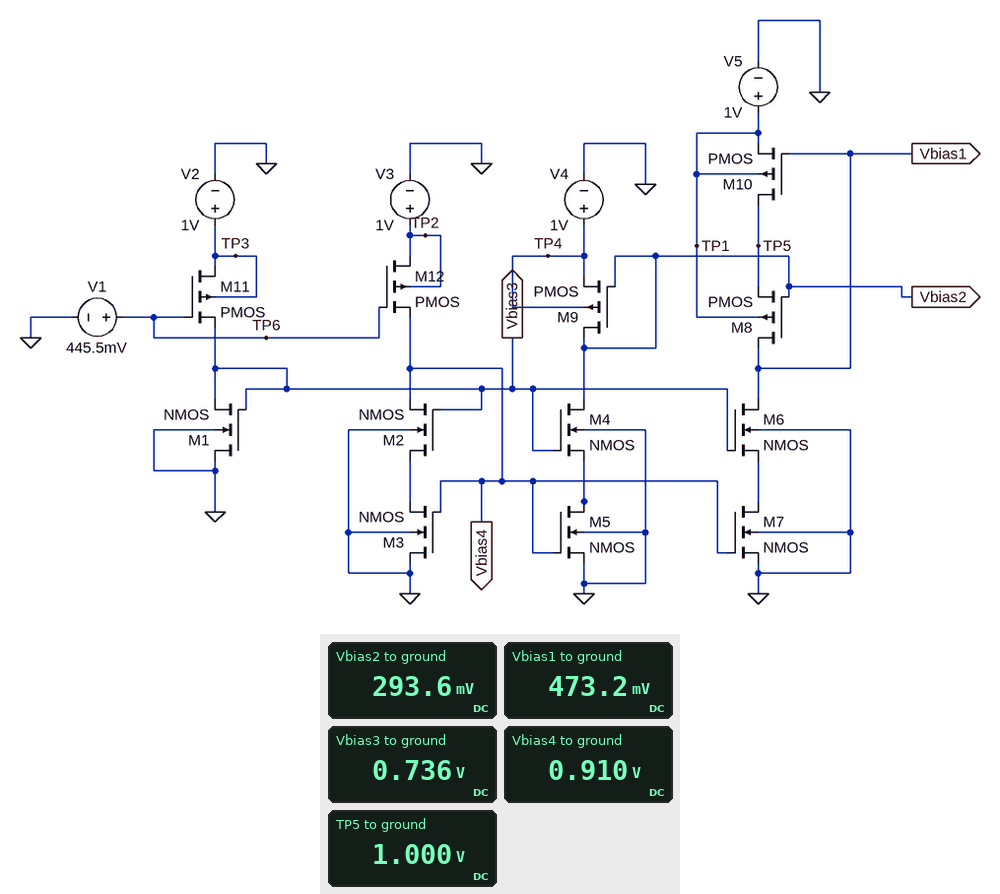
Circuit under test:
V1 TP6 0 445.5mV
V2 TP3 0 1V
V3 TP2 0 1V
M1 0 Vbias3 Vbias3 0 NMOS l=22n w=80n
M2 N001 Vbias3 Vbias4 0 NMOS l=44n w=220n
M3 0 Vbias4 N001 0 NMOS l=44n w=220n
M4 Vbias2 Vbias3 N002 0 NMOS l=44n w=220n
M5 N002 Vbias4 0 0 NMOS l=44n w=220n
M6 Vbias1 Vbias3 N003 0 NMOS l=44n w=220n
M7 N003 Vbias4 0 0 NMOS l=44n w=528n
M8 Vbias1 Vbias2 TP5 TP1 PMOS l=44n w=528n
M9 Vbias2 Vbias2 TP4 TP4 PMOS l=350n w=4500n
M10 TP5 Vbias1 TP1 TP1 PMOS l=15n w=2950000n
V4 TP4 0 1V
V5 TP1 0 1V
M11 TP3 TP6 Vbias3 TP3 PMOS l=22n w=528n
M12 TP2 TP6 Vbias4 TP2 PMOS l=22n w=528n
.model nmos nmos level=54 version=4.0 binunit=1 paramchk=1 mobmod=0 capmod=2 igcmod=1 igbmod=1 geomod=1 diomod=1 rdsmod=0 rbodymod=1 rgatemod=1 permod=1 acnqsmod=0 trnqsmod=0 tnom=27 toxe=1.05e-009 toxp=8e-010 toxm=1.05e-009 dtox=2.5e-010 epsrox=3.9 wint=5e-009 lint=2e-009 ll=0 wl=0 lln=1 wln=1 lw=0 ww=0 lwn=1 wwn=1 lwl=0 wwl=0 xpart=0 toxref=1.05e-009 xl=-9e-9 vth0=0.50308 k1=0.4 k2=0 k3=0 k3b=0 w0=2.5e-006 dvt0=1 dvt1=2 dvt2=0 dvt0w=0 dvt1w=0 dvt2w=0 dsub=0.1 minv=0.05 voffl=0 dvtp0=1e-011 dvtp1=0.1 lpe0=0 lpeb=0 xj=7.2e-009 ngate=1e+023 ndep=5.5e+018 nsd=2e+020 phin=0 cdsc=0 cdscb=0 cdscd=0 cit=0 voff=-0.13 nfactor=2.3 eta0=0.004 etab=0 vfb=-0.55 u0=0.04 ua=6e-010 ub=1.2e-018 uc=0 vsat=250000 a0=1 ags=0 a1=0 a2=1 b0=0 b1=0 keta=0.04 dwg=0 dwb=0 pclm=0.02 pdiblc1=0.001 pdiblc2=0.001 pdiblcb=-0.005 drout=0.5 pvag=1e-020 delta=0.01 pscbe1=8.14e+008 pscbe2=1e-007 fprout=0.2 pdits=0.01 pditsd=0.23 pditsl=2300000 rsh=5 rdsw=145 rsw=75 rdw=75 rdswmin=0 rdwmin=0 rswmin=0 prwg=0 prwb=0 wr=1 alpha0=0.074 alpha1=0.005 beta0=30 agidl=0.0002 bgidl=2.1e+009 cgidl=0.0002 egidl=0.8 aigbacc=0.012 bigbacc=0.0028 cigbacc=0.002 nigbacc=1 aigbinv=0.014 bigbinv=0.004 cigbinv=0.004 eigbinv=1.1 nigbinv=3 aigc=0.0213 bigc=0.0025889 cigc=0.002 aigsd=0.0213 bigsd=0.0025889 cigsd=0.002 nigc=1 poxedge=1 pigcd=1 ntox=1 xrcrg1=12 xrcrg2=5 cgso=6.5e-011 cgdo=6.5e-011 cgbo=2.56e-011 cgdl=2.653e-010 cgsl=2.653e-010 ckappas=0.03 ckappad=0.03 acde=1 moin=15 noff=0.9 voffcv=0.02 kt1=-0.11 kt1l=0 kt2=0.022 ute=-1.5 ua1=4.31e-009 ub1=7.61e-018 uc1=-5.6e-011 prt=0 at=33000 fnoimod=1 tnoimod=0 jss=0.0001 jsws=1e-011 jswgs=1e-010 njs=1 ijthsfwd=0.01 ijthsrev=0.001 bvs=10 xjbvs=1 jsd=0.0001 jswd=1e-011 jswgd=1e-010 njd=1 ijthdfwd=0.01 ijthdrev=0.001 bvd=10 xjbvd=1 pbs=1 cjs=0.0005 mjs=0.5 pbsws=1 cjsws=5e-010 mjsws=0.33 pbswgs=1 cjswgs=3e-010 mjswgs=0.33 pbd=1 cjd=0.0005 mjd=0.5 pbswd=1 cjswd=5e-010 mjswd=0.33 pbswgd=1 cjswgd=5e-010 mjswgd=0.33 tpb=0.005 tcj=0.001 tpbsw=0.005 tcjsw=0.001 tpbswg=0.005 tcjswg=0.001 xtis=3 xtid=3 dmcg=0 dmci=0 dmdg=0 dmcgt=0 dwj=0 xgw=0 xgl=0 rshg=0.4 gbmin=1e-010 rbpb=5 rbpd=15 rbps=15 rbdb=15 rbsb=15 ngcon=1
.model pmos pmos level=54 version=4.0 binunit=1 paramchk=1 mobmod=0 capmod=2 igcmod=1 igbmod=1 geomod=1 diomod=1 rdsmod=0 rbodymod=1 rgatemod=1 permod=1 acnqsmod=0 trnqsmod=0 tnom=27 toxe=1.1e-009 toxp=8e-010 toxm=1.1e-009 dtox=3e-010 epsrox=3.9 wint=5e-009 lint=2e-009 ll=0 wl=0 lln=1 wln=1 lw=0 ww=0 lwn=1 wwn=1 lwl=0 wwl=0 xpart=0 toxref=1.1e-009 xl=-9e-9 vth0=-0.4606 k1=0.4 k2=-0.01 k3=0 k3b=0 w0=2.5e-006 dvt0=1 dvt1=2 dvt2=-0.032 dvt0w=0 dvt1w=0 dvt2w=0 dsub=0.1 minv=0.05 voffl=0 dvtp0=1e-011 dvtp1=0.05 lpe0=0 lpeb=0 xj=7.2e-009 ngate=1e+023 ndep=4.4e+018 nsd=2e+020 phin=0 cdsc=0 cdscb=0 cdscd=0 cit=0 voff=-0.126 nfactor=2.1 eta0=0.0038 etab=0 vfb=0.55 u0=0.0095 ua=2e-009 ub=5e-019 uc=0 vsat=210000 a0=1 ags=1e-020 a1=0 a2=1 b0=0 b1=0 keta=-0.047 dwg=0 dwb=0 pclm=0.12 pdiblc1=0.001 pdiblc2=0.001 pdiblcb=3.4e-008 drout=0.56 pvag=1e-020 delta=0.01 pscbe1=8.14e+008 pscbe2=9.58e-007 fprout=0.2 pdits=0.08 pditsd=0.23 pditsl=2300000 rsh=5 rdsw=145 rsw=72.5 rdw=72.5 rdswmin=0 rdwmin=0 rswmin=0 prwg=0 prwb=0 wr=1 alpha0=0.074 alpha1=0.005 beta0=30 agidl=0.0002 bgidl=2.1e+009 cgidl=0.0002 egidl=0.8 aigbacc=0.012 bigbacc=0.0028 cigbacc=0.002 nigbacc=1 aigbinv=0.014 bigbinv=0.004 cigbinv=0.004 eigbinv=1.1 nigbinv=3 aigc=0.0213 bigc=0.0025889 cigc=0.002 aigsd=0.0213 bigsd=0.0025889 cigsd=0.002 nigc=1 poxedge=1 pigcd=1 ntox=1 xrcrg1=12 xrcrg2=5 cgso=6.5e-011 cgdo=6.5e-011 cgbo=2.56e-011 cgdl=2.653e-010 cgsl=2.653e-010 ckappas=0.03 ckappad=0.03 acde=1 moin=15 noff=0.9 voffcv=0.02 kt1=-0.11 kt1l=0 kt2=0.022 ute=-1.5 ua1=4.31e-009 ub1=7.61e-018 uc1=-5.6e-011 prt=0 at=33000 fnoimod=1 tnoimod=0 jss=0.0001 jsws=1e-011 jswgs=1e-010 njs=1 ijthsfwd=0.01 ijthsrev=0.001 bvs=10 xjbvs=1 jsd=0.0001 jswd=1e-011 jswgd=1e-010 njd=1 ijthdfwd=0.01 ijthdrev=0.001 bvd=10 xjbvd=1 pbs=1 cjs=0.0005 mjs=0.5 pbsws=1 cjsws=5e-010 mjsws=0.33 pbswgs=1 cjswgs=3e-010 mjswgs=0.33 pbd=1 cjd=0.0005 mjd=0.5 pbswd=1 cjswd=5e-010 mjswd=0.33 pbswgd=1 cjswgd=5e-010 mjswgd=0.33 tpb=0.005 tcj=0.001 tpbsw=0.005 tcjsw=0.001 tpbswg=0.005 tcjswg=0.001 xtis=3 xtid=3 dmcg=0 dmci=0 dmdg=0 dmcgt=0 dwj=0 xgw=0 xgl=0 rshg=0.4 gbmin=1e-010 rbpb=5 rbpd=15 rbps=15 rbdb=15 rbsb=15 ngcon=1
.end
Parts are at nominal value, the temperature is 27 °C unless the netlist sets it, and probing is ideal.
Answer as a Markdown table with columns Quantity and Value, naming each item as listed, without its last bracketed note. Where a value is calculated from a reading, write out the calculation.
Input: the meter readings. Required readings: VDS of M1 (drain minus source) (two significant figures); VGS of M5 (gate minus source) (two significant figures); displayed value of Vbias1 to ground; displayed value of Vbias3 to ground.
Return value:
| Quantity | Value |
|---|---|
| VDS of M1 (drain minus source) | 0 V - 736 mV = -740 mV |
| VGS of M5 (gate minus source) | 910 mV = 910 mV |
| displayed value of Vbias1 to ground | 473.2 mV |
| displayed value of Vbias3 to ground | 0.736 V |
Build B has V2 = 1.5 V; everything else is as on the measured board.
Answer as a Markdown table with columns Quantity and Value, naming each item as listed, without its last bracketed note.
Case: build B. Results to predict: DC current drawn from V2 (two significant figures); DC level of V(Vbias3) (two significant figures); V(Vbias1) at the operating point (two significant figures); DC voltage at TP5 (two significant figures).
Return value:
| Quantity | Value |
|---|---|
| DC current drawn from V2 | 250 µA |
| DC level of V(Vbias3) | 1.3 V |
| V(Vbias1) at the operating point | 190 mV |
| DC voltage at TP5 | 1.0 V |
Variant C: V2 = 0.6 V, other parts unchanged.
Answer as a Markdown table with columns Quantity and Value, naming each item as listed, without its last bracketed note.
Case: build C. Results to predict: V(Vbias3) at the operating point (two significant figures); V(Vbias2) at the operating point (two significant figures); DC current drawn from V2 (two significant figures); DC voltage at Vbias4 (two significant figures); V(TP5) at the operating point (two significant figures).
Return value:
| Quantity | Value |
|---|---|
| V(Vbias3) at the operating point | 240 mV |
| V(Vbias2) at the operating point | 720 mV |
| DC current drawn from V2 | 100 nA |
| DC voltage at Vbias4 | 1.0 V |
| V(TP5) at the operating point | 1.0 V |
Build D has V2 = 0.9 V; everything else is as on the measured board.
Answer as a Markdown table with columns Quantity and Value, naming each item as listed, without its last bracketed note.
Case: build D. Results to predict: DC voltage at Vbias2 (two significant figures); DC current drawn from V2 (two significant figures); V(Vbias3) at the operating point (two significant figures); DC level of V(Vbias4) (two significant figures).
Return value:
| Quantity | Value |
|---|---|
| DC voltage at Vbias2 | 420 mV |
| DC current drawn from V2 | 40 µA |
| V(Vbias3) at the operating point | 570 mV |
| DC level of V(Vbias4) | 970 mV |
